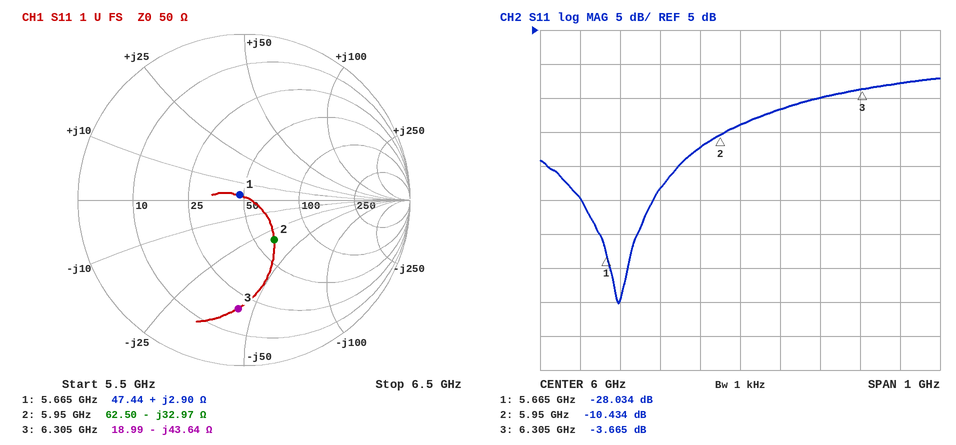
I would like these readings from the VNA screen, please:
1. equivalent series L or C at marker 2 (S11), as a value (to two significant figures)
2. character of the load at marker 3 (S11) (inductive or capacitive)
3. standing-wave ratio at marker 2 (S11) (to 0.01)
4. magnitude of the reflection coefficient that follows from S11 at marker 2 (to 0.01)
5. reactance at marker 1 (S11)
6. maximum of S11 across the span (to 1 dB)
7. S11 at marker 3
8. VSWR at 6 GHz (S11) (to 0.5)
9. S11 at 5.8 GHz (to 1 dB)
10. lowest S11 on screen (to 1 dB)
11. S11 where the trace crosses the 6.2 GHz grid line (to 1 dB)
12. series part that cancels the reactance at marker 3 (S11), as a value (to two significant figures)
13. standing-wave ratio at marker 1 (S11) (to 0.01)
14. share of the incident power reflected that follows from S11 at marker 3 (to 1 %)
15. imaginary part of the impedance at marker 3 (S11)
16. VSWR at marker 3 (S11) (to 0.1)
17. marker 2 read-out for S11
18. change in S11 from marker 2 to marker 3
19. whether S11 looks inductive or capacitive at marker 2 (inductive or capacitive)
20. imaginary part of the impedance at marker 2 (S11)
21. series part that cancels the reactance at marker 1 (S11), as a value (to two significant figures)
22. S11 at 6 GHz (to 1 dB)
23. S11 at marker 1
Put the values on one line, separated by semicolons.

810 fF; capacitive; 1.86; 0.30; +2.90 Ω; -2 dB; -3.665 dB; 2.0; -18 dB; -35 dB; -5 dB; 1.1 nH; 1.08; 43 %; -43.64 Ω; 4.8; -10.434 dB; 6.769 dB; capacitive; -32.97 Ω; 9.7 pF; -9 dB; -28.034 dB
